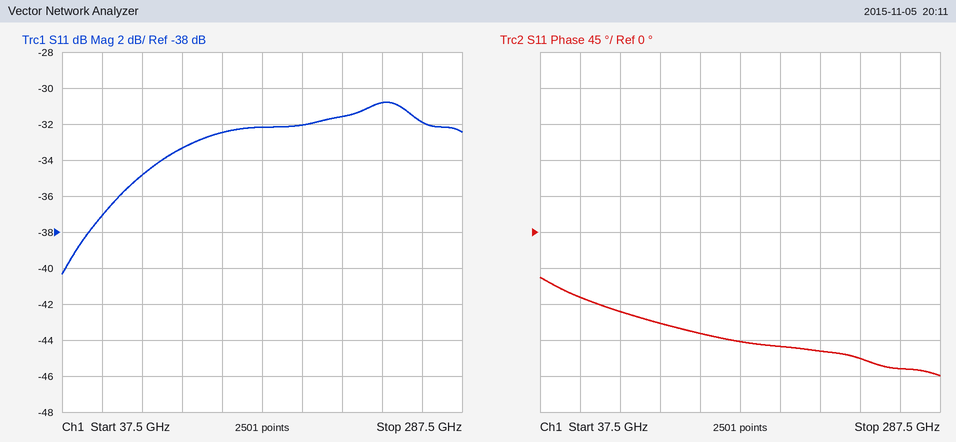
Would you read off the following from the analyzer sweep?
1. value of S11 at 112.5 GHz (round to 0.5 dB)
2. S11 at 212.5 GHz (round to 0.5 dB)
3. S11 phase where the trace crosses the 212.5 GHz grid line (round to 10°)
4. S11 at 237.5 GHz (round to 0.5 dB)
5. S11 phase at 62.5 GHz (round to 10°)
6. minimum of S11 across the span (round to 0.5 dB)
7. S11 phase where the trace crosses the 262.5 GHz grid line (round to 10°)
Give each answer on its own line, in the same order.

-33.5 dB
-31.5 dB
-150°
-31.0 dB
-80°
-40.5 dB
-170°
